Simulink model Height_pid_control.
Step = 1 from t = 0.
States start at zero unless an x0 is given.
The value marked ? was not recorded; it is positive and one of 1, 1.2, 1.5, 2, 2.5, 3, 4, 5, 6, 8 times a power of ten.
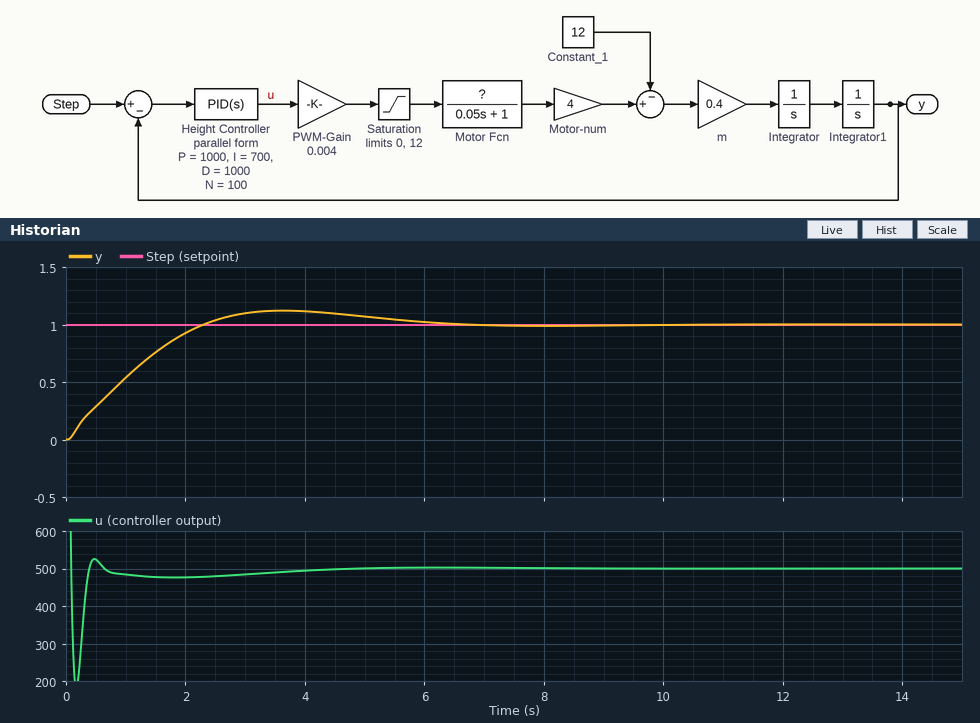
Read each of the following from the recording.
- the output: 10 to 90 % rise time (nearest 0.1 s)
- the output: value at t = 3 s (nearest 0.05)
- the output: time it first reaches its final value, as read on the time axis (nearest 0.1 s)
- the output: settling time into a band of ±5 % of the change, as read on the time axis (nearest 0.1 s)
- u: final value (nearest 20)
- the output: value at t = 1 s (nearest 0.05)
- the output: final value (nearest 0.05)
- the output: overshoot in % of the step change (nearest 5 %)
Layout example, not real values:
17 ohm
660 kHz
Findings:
1.7 s
1.10
2.3 s
5.4 s
500
0.55
1.00
10 %
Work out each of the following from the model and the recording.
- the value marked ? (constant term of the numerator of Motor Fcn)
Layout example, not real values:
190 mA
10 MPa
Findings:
1.5
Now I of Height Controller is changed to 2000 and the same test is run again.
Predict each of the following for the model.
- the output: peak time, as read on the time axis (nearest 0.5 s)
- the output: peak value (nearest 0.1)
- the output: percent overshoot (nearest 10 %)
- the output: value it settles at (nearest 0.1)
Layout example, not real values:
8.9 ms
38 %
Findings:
2.0 s
1.4
40 %
1.0
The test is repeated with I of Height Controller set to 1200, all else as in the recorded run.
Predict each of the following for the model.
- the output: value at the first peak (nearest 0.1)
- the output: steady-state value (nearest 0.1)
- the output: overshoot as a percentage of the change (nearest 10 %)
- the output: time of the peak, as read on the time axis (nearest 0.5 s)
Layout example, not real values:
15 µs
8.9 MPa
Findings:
1.2
1.0
20 %
2.5 s
